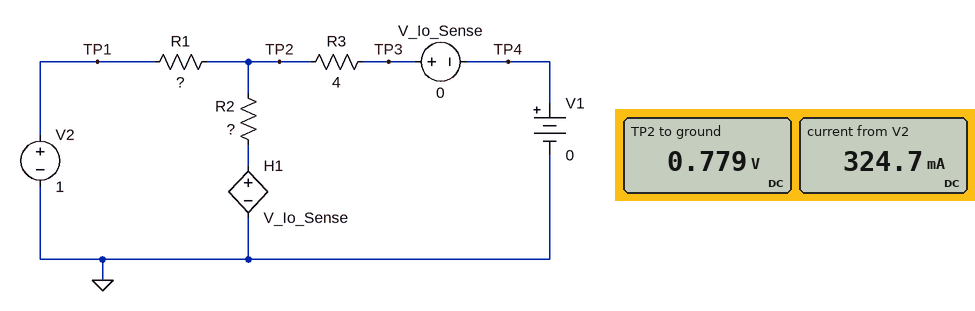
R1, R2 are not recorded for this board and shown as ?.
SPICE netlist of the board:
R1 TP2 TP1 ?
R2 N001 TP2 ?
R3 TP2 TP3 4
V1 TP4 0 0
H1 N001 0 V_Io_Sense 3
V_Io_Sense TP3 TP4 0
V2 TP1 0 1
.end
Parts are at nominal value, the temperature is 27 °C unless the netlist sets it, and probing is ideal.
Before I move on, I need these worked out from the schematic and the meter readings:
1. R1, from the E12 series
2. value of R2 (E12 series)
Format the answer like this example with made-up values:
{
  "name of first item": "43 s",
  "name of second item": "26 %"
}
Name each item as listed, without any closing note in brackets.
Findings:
{
  "R1, from the E12 series": "0.68 Ω",
  "value of R2": "1.5 Ω"
}
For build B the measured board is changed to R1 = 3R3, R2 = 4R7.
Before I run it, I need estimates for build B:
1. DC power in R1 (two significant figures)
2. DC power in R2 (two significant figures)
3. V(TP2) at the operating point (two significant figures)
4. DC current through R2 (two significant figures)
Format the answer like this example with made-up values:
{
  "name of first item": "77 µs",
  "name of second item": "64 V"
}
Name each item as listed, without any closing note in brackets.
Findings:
{
  "DC power in R1": "76 mW",
  "DC power in R2": "3.3 mW",
  "V(TP2) at the operating point": "500 mV",
  "DC current through R2": "27 mA"
}
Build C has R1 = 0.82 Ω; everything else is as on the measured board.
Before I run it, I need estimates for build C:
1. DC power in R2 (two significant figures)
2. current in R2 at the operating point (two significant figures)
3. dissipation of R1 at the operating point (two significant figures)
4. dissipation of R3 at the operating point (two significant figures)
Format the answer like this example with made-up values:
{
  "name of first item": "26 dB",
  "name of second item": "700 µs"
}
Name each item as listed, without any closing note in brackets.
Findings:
{
  "DC power in R2": "23 mW",
  "current in R2 at the operating point": "120 mA",
  "dissipation of R1 at the operating point": "79 mW",
  "dissipation of R3 at the operating point": "140 mW"
}
